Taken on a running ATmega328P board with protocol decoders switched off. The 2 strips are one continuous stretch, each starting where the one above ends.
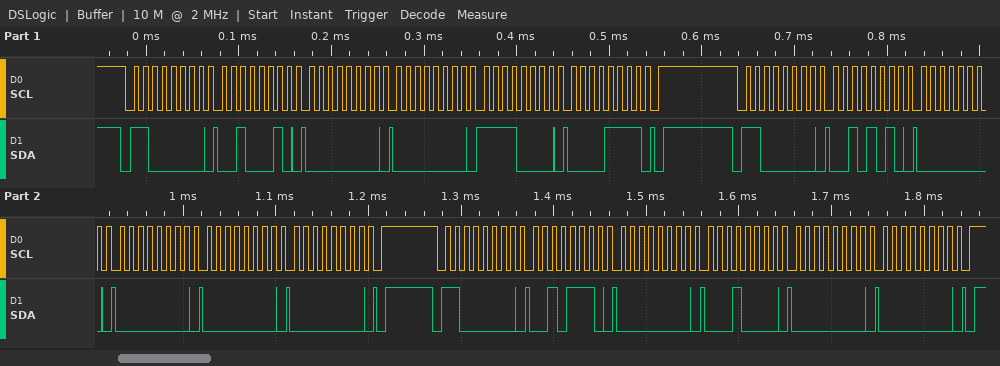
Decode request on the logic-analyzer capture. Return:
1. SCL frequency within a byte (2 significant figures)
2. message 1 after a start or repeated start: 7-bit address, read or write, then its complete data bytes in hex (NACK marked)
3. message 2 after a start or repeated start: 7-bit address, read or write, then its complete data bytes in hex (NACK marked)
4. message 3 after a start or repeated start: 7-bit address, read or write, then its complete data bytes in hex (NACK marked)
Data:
100 kHz
0x60 write: 22 00 00 F0 0F
0x60 write: 2A 00 00 00 00
0x60 write: 2E 00 10 00 00
